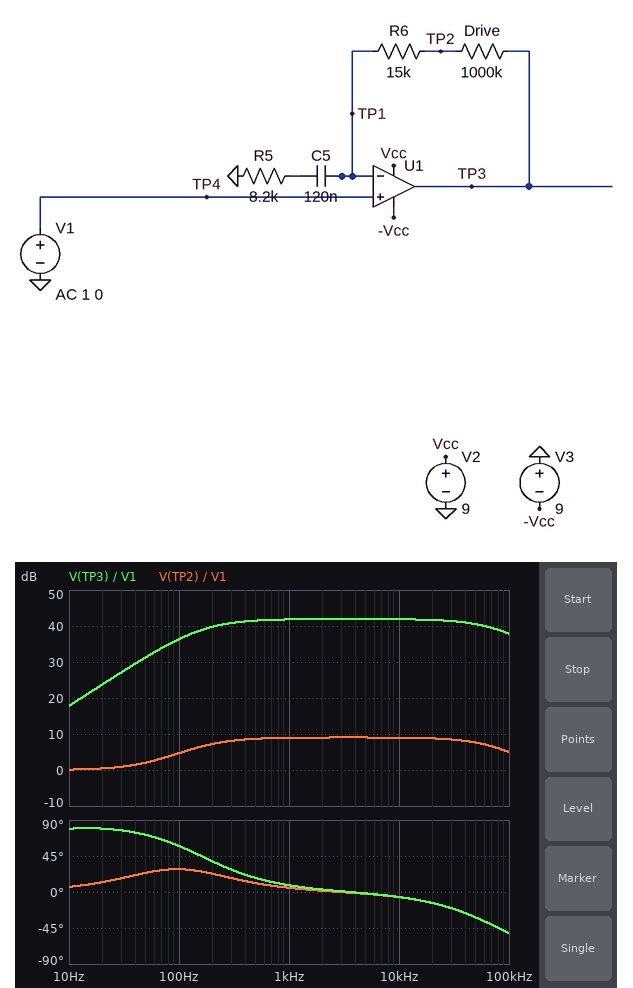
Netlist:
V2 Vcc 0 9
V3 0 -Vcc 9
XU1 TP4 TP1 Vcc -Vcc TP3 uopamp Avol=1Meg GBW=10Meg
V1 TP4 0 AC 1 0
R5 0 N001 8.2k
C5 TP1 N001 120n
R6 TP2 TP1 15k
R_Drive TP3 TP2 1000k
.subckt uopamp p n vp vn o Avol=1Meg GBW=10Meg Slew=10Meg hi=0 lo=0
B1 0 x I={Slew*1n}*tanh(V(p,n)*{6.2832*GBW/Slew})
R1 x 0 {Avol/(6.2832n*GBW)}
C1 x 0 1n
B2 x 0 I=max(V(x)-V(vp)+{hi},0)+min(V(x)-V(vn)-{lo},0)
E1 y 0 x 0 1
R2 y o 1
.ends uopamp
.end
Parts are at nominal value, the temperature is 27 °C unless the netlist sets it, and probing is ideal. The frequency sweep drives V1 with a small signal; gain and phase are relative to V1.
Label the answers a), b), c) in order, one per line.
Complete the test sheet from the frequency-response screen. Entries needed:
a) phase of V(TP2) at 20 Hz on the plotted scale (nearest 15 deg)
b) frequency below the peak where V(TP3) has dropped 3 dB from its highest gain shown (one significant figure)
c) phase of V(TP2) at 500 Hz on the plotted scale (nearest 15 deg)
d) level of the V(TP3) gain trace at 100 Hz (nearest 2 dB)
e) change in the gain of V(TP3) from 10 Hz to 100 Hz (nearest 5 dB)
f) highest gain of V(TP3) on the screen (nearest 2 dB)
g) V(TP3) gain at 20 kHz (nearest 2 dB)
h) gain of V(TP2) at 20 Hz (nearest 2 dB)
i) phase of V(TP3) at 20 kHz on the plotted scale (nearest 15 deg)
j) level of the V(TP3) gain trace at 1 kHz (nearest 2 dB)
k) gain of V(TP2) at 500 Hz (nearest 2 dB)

a) 15 deg
b) 200 Hz
c) 15 deg
d) 36 dB
e) 20 dB
f) 42 dB
g) 42 dB
h) 0 dB
i) -15 deg
j) 42 dB
k) 8 dB
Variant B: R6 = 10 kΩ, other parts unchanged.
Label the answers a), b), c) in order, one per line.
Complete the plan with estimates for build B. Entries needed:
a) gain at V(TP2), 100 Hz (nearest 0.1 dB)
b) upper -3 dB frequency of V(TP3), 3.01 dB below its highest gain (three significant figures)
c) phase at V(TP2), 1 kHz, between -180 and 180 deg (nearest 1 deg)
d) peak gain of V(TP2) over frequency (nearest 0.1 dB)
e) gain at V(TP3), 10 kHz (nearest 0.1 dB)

a) 3.2 dB
b) 80.7 kHz
c) 4 deg
d) 6.9 dB
e) 41.8 dB
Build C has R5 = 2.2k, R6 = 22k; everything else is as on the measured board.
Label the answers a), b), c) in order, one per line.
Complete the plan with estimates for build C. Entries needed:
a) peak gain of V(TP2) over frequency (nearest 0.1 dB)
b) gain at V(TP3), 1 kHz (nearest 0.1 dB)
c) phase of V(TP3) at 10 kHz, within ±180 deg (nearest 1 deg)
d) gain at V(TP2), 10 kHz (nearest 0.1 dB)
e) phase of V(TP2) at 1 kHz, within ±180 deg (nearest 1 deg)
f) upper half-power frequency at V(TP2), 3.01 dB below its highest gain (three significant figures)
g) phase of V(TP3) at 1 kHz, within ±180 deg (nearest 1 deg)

a) 20.8 dB
b) 52.2 dB
c) -22 deg
d) 20.2 dB
e) 26 deg
f) 22.1 kHz
g) 29 deg
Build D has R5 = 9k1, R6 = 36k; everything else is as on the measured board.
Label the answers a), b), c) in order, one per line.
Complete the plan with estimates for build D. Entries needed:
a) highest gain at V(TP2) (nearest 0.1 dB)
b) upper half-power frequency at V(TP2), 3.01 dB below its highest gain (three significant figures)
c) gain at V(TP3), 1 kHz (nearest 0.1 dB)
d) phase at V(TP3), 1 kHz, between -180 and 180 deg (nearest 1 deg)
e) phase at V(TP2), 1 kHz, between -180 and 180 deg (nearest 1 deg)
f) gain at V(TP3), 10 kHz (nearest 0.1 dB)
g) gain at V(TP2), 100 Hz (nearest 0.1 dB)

a) 13.9 dB
b) 87.2 kHz
c) 41.1 dB
d) 8 deg
e) 6 deg
f) 41.2 dB
g) 9.3 dB
